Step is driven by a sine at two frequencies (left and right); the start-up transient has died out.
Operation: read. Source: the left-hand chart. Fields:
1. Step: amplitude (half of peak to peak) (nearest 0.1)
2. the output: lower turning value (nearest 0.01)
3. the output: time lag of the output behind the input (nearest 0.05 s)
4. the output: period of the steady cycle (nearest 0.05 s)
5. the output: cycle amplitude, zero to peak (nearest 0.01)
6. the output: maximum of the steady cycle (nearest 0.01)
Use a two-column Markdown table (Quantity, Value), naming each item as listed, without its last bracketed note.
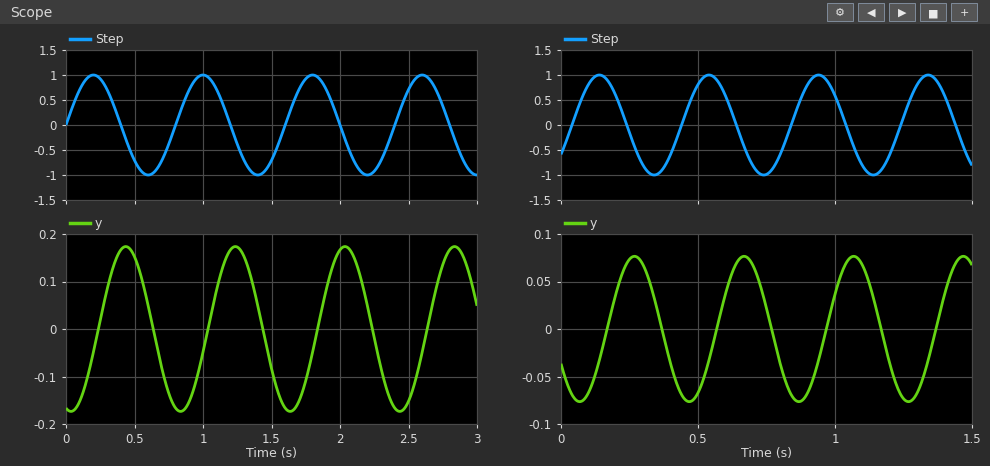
| Quantity | Value |
|---|---|
| Step: amplitude (half of peak to peak) | 1.0 |
| the output: lower turning value | -0.17 |
| the output: time lag of the output behind the input | 0.25 s |
| the output: period of the steady cycle | 0.80 s |
| the output: cycle amplitude, zero to peak | 0.17 |
| the output: maximum of the steady cycle | 0.17 |
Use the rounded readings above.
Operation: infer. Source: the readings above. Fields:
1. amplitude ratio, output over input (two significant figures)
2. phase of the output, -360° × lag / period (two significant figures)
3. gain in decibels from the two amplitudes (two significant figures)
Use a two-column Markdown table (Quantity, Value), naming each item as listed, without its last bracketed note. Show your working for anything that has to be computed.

| Quantity | Value |
|---|---|
| amplitude ratio, output over input | 0.17 / 1 = 0.17 |
| phase of the output, -360° × lag / period | -360 × 0.25 / 0.8 = -110° |
| gain in decibels from the two amplitudes | 20 log10(0.17 / 1) = -15 dB |
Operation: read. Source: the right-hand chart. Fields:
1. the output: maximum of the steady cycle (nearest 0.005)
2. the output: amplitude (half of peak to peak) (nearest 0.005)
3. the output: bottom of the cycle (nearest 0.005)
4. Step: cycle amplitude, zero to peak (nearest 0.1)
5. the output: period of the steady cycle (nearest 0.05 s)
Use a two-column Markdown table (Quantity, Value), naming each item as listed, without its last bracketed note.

| Quantity | Value |
|---|---|
| the output: maximum of the steady cycle | 0.075 |
| the output: amplitude (half of peak to peak) | 0.075 |
| the output: bottom of the cycle | -0.075 |
| Step: cycle amplitude, zero to peak | 1.0 |
| the output: period of the steady cycle | 0.40 s |
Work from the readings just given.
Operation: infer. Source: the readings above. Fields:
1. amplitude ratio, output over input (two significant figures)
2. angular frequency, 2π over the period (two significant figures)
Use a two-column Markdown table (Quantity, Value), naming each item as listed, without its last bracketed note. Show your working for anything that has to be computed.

| Quantity | Value |
|---|---|
| amplitude ratio, output over input | 0.075 / 1 = 0.075 |
| angular frequency, 2π over the period | 2π / 0.4 = 16 rad/s |
